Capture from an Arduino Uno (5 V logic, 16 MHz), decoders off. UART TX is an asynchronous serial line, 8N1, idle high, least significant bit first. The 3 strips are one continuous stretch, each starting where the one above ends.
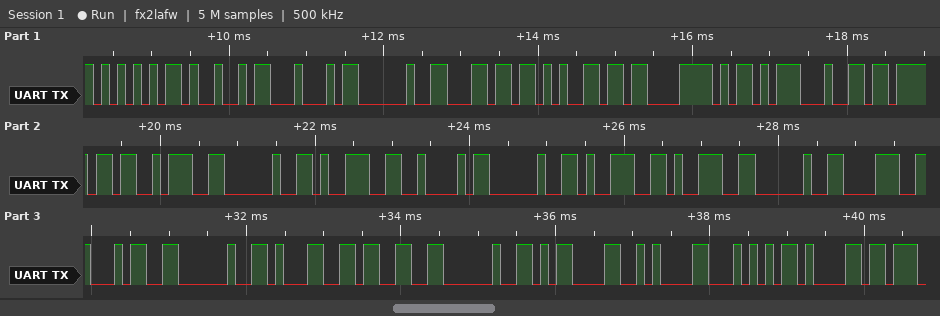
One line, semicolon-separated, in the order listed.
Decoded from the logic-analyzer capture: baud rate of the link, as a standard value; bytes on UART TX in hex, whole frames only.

9600 baud; 55 49 44 20 6C 65 C3 AD 64 6F 3A 20 39 42 20 39 39 20 38 34 20 31 33 20 0D 0A 54 61
